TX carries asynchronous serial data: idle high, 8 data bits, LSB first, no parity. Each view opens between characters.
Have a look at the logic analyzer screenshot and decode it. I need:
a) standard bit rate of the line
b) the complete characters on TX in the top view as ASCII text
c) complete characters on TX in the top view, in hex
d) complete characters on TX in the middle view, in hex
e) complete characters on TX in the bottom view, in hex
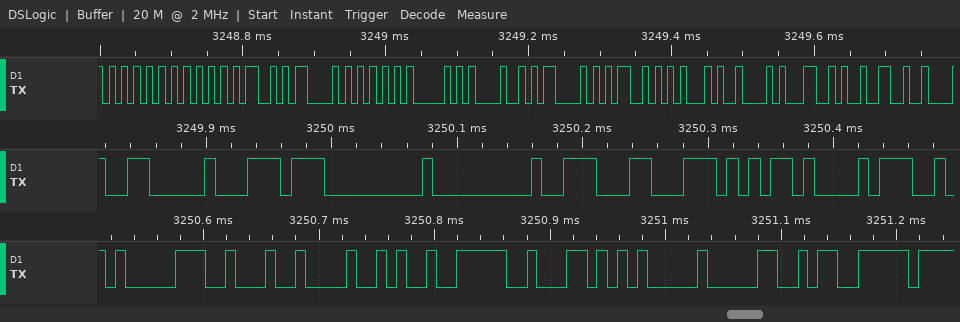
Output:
115200 baud
"UUMCUPHCMEBL2"
55, 55, 4D, 43, 55, 50, 48, 43, 4D, 45, 42, 4C, 32
06, DC, 00, 00, 8E, 5C, 0B
C1, 22, 48, F2, 62, 05, 30, F3
